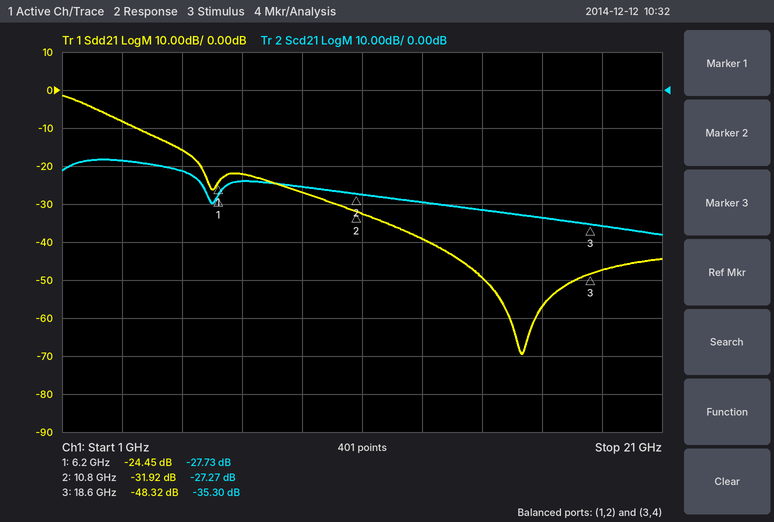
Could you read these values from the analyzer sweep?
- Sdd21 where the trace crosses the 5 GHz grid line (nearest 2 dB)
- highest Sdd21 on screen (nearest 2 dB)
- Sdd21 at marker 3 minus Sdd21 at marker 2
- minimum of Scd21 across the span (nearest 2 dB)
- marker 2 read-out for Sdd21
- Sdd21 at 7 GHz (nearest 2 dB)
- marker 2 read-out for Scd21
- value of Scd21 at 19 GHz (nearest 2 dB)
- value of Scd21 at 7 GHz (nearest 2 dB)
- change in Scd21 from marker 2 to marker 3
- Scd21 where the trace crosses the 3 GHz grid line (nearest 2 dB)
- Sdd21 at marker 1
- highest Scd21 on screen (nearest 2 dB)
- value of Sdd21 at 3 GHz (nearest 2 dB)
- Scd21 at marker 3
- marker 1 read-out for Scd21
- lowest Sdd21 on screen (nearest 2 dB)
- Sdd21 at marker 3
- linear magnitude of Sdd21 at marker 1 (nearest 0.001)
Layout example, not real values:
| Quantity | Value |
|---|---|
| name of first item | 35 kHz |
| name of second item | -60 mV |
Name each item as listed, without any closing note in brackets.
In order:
| Quantity | Value |
|---|---|
| Sdd21 where the trace crosses the 5 GHz grid line | -16 dB |
| highest Sdd21 on screen | -2 dB |
| Sdd21 at marker 3 minus Sdd21 at marker 2 | -16.40 dB |
| minimum of Scd21 across the span | -38 dB |
| marker 2 read-out for Sdd21 | -31.92 dB |
| Sdd21 at 7 GHz | -22 dB |
| marker 2 read-out for Scd21 | -27.27 dB |
| value of Scd21 at 19 GHz | -36 dB |
| value of Scd21 at 7 GHz | -24 dB |
| change in Scd21 from marker 2 to marker 3 | -8.03 dB |
| Scd21 where the trace crosses the 3 GHz grid line | -18 dB |
| Sdd21 at marker 1 | -24.45 dB |
| highest Scd21 on screen | -18 dB |
| value of Sdd21 at 3 GHz | -8 dB |
| Scd21 at marker 3 | -35.30 dB |
| marker 1 read-out for Scd21 | -27.73 dB |
| lowest Sdd21 on screen | -70 dB |
| Sdd21 at marker 3 | -48.32 dB |
| linear magnitude of Sdd21 at marker 1 | 0.060 |
